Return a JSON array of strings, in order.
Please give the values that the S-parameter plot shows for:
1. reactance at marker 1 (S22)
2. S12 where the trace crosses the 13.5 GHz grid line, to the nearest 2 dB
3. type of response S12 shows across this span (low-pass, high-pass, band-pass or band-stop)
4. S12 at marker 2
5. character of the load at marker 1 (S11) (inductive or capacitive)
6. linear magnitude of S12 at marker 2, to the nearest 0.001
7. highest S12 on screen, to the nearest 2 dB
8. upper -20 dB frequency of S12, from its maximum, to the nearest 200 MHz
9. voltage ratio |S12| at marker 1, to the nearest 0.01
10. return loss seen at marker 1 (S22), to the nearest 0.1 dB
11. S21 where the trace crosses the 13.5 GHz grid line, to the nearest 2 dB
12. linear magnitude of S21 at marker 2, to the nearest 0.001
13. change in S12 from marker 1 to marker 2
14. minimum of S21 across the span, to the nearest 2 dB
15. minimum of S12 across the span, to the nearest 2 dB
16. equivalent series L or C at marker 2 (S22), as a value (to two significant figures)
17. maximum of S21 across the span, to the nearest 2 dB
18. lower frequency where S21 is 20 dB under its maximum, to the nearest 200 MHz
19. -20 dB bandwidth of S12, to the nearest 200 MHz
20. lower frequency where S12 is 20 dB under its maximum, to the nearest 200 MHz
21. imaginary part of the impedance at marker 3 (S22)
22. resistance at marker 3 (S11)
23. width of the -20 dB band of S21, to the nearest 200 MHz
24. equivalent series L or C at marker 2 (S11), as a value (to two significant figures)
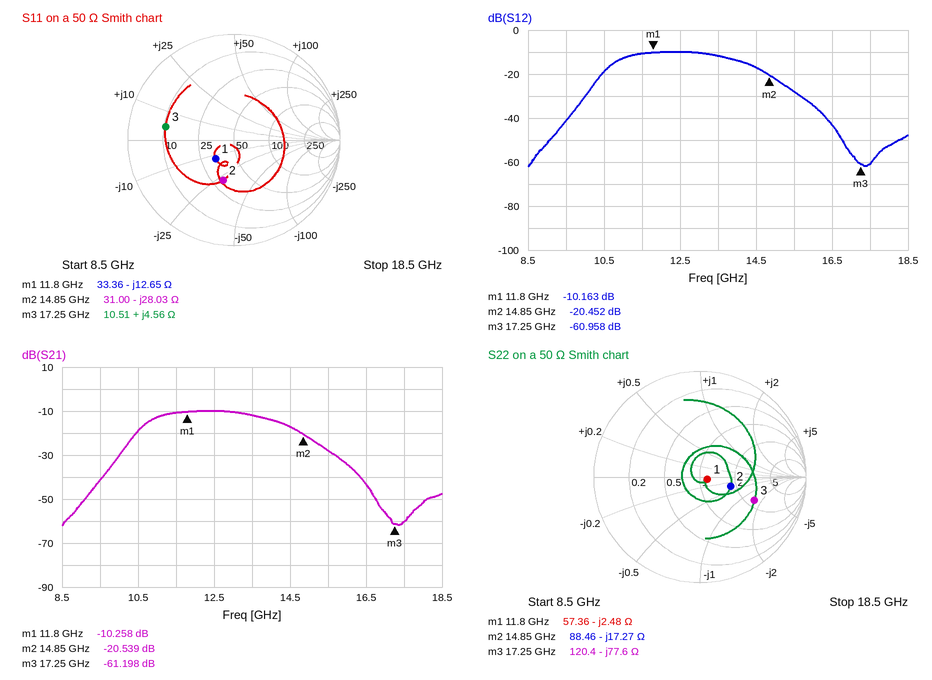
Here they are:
["-2.48 Ω", "-12 dB", "band-pass", "-20.452 dB", "capacitive", "0.095", "-10 dB", "15.6 GHz", "0.31", "22.8 dB", "-12 dB", "0.094", "-10.289 dB", "-62 dB", "-62 dB", "620 fF", "-10 dB", "10.0 GHz", "5.6 GHz", "10.0 GHz", "-77.6 Ω", "10.51 Ω", "5.6 GHz", "380 fF"]
